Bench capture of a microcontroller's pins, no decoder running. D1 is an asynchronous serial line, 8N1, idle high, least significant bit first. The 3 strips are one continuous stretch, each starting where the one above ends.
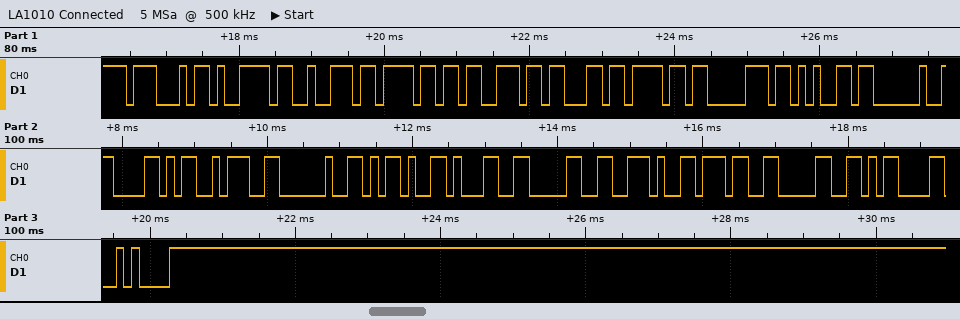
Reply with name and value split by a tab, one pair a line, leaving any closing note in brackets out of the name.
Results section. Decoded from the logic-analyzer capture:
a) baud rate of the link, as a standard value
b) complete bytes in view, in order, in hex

baud rate of the link, as a standard value	9600 baud
complete bytes in view, in order, in hex	47 79 72 6F 73 63 6F 70 65 20 58 3A 20 2D 31 30 2E 37 30 0D 0A
